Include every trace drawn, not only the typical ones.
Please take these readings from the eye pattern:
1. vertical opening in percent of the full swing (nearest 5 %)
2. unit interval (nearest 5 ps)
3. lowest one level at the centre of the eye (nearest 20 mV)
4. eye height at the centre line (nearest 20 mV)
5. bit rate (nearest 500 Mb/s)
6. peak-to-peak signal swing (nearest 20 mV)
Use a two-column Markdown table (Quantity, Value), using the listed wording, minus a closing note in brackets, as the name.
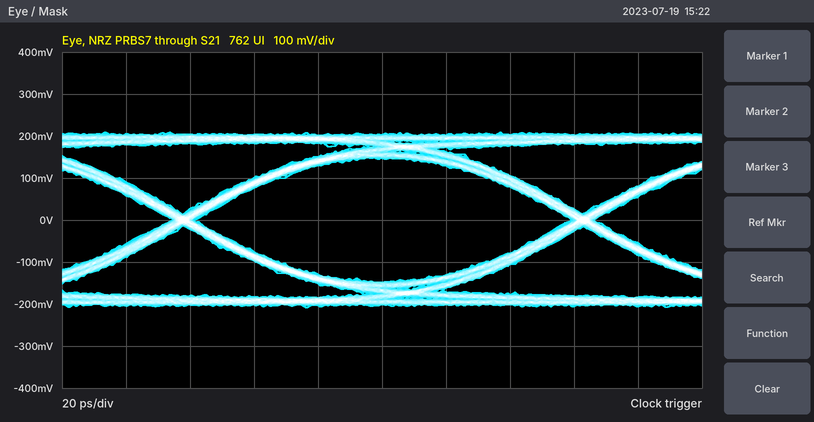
| Quantity | Value |
|---|---|
| vertical opening in percent of the full swing | 70 % |
| unit interval | 125 ps |
| lowest one level at the centre of the eye | 140 mV |
| eye height at the centre line | 300 mV |
| bit rate | 8.0 Gb/s |
| peak-to-peak signal swing | 420 mV |
